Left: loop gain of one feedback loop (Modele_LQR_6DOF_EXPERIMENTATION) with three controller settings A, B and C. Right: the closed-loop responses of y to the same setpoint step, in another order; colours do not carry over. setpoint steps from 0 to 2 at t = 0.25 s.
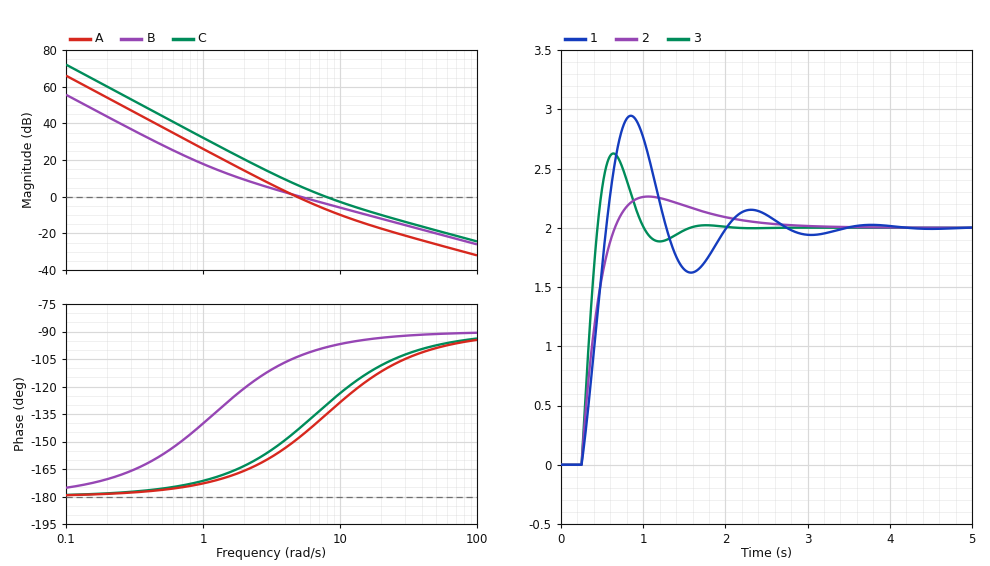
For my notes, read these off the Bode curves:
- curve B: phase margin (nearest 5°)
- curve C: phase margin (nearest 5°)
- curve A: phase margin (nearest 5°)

75°
50°
30°
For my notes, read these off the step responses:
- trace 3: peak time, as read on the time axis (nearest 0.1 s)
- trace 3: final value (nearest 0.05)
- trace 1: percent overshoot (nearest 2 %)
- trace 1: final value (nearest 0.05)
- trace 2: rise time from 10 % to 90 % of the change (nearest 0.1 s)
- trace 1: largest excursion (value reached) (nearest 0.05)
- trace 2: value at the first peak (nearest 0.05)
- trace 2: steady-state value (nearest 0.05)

0.6 s
2.00
48 %
2.00
0.3 s
2.95
2.25
2.00
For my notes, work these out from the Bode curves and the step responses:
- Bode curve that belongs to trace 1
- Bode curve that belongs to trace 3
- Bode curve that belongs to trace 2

A
C
B
